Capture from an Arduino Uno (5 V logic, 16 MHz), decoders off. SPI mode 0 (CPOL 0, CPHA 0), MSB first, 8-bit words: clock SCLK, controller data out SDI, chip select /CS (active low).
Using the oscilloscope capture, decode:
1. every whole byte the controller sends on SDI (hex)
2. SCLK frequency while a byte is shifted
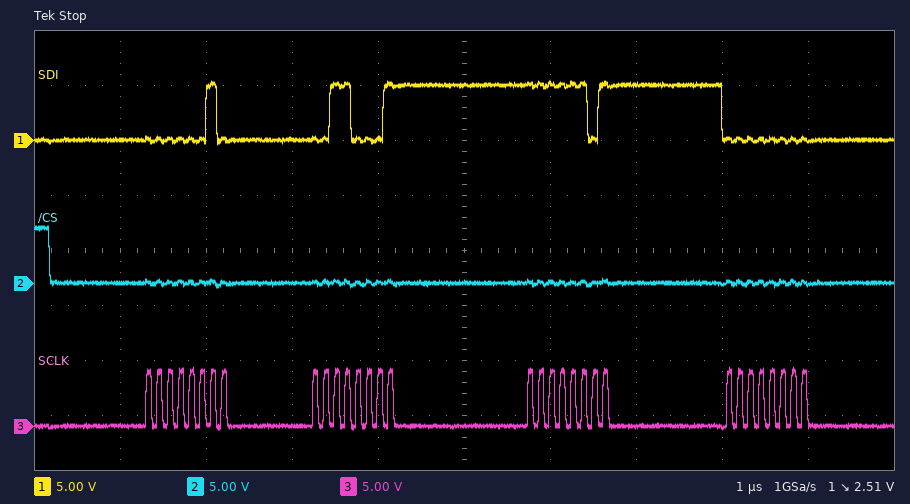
02 31 FD 00
8 MHz
